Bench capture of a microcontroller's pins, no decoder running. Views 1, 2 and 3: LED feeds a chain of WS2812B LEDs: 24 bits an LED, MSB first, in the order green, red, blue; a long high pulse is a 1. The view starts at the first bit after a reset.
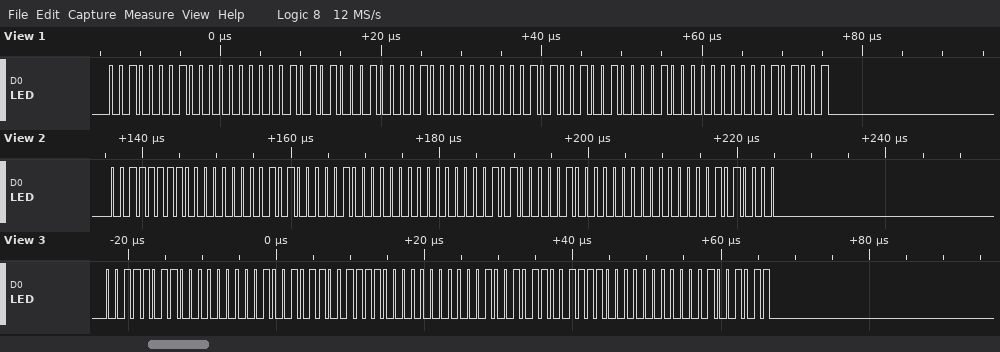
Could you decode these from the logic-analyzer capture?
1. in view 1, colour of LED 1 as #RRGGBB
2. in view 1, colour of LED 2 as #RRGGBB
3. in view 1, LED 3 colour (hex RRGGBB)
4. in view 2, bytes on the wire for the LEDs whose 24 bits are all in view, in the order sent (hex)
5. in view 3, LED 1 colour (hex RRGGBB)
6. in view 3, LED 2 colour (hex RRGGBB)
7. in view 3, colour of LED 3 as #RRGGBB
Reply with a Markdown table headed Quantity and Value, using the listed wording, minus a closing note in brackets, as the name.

| Quantity | Value |
|---|---|
| in view 1, colour of LED 1 as #RRGGBB | #00212A |
| in view 1, colour of LED 2 as #RRGGBB | #002129 |
| in view 1, LED 3 colour | #002129 |
| in view 2, bytes on the wire for the LEDs whose 24 bits are all in view, in the order sent | 3F 00 50 40 00 50 40 00 50 |
| in view 3, LED 1 colour | #003B4B |
| in view 3, LED 2 colour | #003C4B |
| in view 3, colour of LED 3 as #RRGGBB | #003C4B |
